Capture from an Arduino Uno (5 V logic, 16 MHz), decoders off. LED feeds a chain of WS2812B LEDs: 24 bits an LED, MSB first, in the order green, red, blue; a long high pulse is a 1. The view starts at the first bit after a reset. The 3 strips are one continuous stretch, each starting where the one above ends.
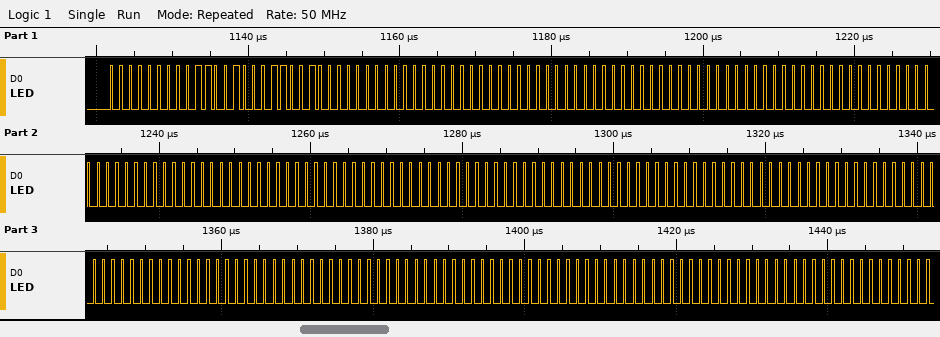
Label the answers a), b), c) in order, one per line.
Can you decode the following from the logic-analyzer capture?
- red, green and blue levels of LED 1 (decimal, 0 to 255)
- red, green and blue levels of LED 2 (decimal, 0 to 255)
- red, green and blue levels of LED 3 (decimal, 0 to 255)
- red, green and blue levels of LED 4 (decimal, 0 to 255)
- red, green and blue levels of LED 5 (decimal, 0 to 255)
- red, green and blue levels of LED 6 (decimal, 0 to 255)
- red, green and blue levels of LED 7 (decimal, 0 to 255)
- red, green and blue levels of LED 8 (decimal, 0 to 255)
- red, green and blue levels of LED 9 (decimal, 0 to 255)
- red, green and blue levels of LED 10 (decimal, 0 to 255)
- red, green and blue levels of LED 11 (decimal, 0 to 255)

a) 100, 0, 100
b) 0, 0, 0
c) 0, 0, 0
d) 0, 0, 0
e) 0, 0, 0
f) 0, 0, 0
g) 0, 0, 0
h) 0, 0, 0
i) 0, 0, 0
j) 0, 0, 0
k) 0, 0, 0
